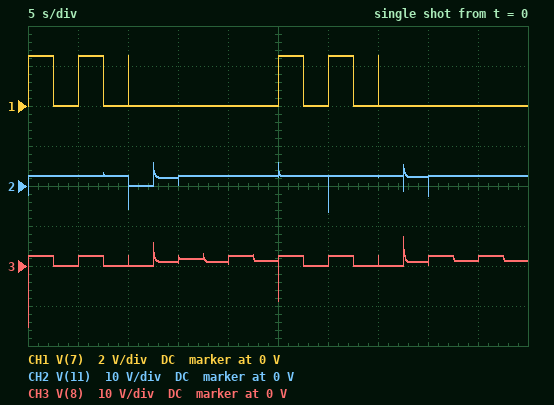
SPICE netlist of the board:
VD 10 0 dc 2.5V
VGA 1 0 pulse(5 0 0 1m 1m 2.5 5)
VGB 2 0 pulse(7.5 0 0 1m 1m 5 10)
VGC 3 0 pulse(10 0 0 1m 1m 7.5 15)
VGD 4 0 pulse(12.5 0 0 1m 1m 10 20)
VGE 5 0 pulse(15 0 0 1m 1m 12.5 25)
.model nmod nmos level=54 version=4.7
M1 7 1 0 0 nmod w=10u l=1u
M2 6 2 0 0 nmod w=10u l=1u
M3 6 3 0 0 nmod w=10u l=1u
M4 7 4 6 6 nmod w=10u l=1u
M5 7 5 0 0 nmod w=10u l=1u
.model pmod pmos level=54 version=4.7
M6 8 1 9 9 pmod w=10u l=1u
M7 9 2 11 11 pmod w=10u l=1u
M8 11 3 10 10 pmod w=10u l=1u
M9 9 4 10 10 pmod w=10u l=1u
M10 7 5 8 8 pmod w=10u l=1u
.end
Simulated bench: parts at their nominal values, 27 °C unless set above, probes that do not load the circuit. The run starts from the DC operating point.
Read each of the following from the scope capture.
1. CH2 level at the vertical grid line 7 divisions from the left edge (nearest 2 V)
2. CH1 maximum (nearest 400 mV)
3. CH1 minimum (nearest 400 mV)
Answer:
2 V
2.4 V
0 V
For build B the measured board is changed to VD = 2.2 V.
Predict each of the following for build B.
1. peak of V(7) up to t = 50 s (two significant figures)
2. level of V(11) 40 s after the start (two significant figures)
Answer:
2.2 V
1.9 V
